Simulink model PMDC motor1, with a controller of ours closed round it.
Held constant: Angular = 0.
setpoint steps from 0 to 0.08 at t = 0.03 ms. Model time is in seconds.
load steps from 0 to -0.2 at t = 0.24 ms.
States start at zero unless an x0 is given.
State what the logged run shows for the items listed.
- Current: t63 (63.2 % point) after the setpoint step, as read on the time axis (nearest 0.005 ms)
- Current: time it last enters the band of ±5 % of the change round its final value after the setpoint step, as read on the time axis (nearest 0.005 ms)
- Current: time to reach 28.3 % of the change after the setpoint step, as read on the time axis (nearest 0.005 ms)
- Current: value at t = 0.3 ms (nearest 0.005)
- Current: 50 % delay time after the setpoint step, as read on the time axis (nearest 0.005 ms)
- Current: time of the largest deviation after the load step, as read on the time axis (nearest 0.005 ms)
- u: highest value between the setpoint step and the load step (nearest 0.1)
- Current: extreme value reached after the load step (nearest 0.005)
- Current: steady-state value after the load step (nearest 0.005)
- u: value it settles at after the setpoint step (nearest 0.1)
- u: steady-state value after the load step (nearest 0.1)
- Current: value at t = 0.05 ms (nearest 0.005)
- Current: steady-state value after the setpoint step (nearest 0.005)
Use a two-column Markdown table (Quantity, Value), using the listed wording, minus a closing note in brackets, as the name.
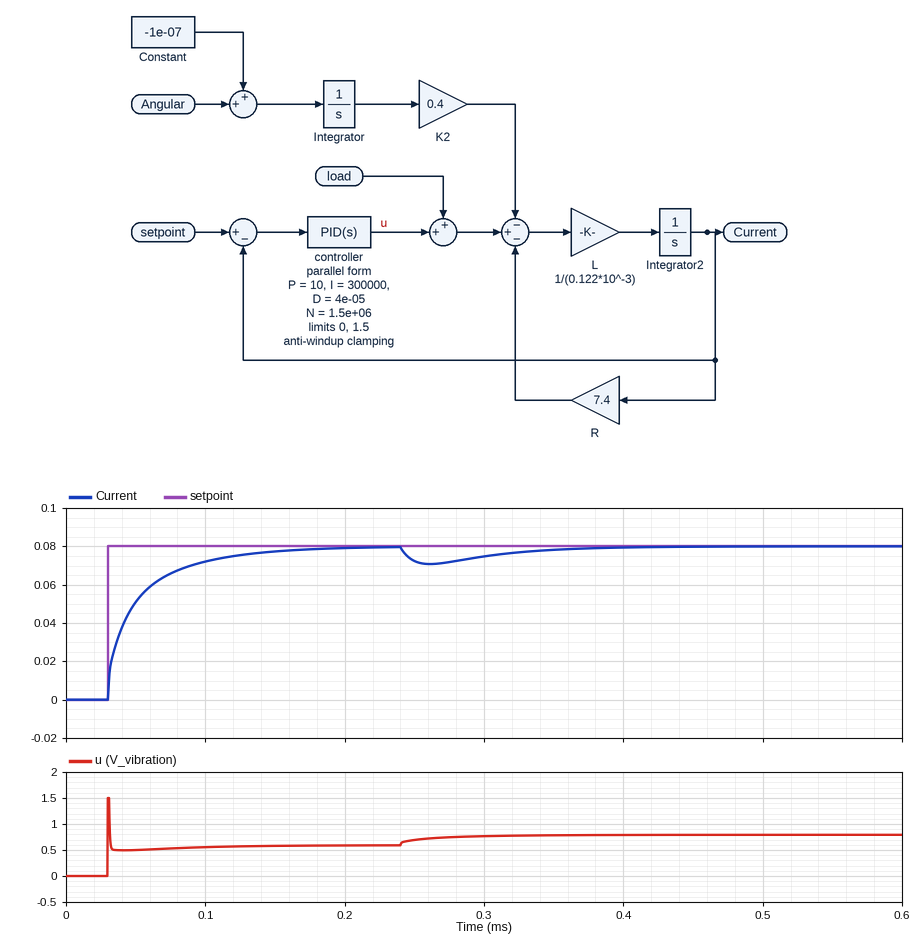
| Quantity | Value |
|---|---|
| Current: t63 (63.2 % point) after the setpoint step, as read on the time axis | 0.050 ms |
| Current: time it last enters the band of ±5 % of the change round its final value after the setpoint step, as read on the time axis | 0.130 ms |
| Current: time to reach 28.3 % of the change after the setpoint step, as read on the time axis | 0.035 ms |
| Current: value at t = 0.3 ms | 0.075 |
| Current: 50 % delay time after the setpoint step, as read on the time axis | 0.040 ms |
| Current: time of the largest deviation after the load step, as read on the time axis | 0.260 ms |
| u: highest value between the setpoint step and the load step | 1.5 |
| Current: extreme value reached after the load step | 0.070 |
| Current: steady-state value after the load step | 0.080 |
| u: value it settles at after the setpoint step | 0.6 |
| u: steady-state value after the load step | 0.8 |
| Current: value at t = 0.05 ms | 0.050 |
| Current: steady-state value after the setpoint step | 0.080 |
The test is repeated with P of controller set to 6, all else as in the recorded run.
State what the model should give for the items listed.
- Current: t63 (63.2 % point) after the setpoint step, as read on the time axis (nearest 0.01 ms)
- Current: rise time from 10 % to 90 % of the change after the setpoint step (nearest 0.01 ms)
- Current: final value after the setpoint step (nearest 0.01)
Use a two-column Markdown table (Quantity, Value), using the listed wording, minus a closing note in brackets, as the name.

| Quantity | Value |
|---|---|
| Current: t63 (63.2 % point) after the setpoint step, as read on the time axis | 0.06 ms |
| Current: rise time from 10 % to 90 % of the change after the setpoint step | 0.06 ms |
| Current: final value after the setpoint step | 0.08 |
